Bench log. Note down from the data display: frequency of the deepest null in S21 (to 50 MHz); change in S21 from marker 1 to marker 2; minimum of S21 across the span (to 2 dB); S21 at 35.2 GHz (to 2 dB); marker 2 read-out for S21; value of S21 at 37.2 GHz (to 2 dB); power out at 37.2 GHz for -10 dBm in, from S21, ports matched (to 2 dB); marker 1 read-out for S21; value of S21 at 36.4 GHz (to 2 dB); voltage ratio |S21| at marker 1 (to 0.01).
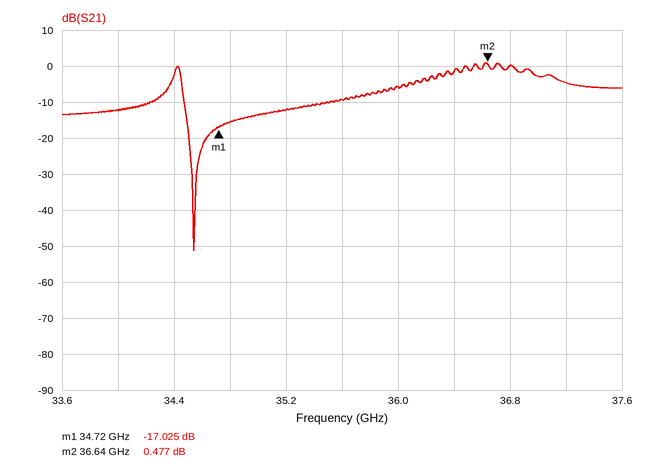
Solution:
34.55 GHz
17.502 dB
-52 dB
-12 dB
0.477 dB
-4 dB
-14 dBm
-17.025 dB
-2 dB
0.14
